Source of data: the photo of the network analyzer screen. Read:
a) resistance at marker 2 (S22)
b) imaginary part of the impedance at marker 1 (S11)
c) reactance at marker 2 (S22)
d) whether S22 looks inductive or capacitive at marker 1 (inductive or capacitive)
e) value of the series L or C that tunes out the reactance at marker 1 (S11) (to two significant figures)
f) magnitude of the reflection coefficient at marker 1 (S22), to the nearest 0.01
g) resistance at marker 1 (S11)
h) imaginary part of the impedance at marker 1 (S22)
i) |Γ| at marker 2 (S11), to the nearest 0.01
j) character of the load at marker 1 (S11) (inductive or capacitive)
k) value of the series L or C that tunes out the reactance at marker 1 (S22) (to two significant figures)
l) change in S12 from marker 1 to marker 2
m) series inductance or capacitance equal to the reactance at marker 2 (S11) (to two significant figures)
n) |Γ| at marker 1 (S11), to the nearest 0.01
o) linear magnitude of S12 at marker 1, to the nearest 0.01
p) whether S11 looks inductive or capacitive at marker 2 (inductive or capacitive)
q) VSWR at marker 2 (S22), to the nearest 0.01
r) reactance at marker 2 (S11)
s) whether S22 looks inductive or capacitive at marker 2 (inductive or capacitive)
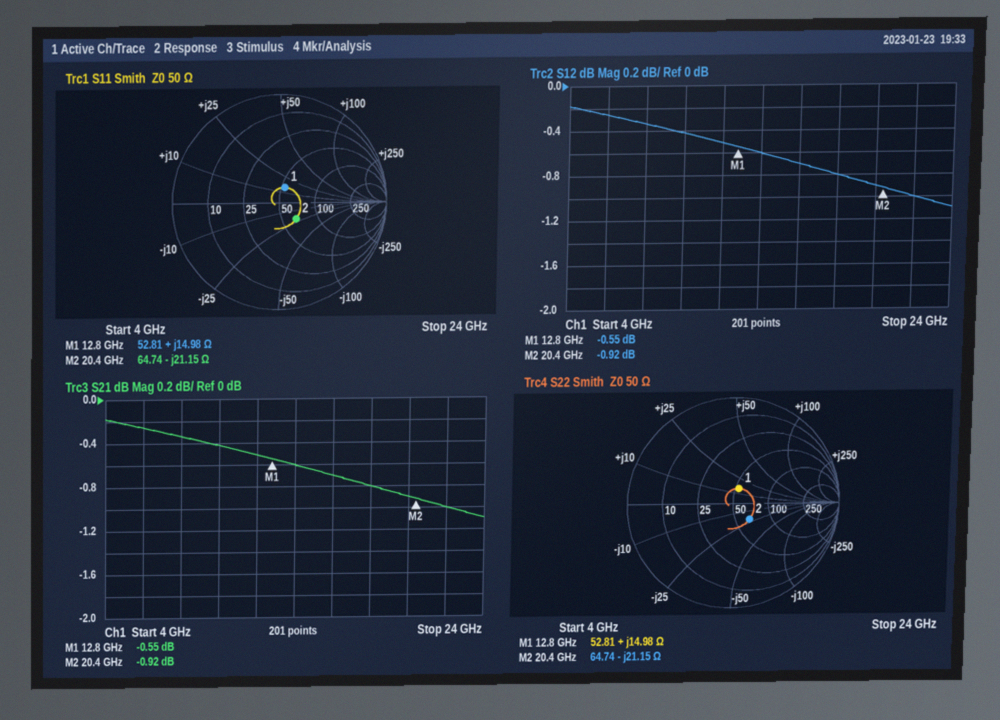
64.74 Ω
+14.98 Ω
-21.15 Ω
inductive
830 fF
0.15
52.81 Ω
+14.98 Ω
0.22
inductive
830 fF
-0.37 dB
370 fF
0.15
0.94
capacitive
1.57
-21.15 Ω
capacitive
